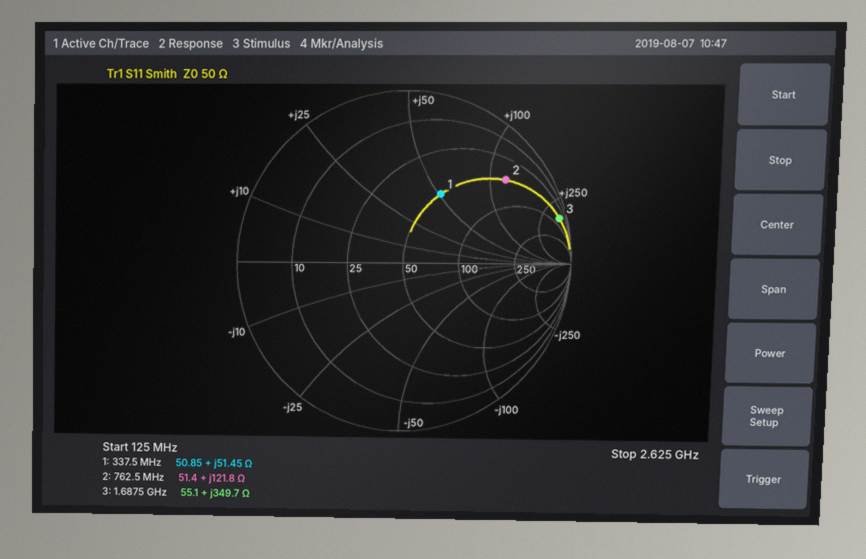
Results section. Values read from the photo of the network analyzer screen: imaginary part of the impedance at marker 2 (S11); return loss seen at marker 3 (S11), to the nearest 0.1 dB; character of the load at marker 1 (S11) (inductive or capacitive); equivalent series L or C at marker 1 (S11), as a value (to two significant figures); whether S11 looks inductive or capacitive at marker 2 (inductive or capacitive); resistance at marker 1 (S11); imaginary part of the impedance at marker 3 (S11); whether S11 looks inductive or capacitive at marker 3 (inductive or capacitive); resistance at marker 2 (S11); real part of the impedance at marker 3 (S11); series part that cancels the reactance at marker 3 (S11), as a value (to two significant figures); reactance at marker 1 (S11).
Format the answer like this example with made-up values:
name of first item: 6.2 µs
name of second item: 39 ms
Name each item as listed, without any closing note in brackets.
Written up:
imaginary part of the impedance at marker 2: +121.8 Ω
return loss seen at marker 3 (S11), to the nearest 0.1 dB: 0.4 dB
character of the load at marker 1 (S11): inductive
equivalent series L or C at marker 1 (S11), as a value: 24 nH
whether S11 looks inductive or capacitive at marker 2: inductive
resistance at marker 1: 50.85 Ω
imaginary part of the impedance at marker 3: +349.7 Ω
whether S11 looks inductive or capacitive at marker 3: inductive
resistance at marker 2: 51.4 Ω
real part of the impedance at marker 3: 55.1 Ω
series part that cancels the reactance at marker 3 (S11), as a value: 270 fF
reactance at marker 1: +51.45 Ω
